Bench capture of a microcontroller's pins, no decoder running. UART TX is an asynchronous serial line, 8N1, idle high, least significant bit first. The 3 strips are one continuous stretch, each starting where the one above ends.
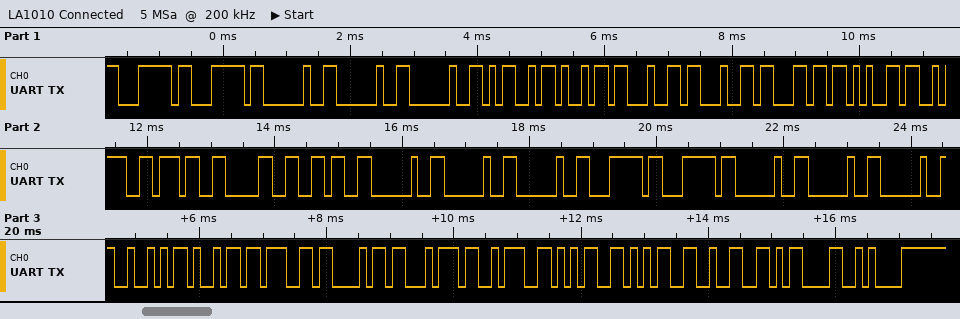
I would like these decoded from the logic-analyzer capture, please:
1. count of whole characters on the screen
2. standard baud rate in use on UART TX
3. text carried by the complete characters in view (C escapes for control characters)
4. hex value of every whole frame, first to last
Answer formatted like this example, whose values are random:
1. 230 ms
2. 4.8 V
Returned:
1. 34
2. 9600 baud
3. "||   Middle:706   ||   Right:552\r\n"
4. 0x7C 0x7C 0x20 0x20 0x20 0x4D 0x69 0x64 0x64 0x6C 0x65 0x3A 0x37 0x30 0x36 0x20 0x20 0x20 0x7C 0x7C 0x20 0x20 0x20 0x52 0x69 0x67 0x68 0x74 0x3A 0x35 0x35 0x32 0x0D 0x0A
